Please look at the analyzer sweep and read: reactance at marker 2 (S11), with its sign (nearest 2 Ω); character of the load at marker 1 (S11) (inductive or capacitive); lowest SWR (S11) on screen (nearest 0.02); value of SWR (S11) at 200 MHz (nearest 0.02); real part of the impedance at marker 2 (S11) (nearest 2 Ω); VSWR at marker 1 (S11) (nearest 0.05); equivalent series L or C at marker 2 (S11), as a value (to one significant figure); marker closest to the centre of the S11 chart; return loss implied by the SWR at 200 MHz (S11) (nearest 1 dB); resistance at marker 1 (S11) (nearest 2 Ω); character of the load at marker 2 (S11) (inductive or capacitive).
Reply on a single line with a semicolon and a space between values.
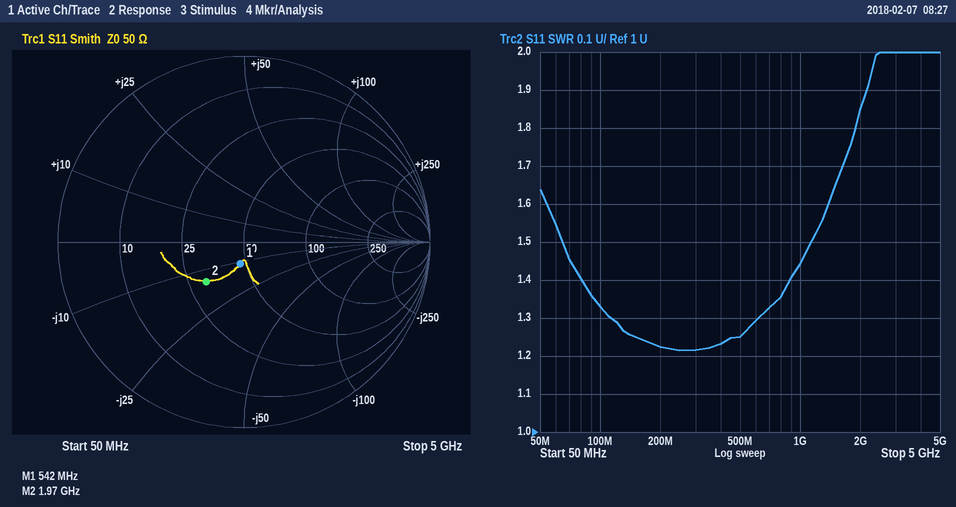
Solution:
-14 Ω; capacitive; 1.22; 1.22; 30 Ω; 1.25; 6 pF; marker 1; 20 dB; 46 Ω; capacitive
